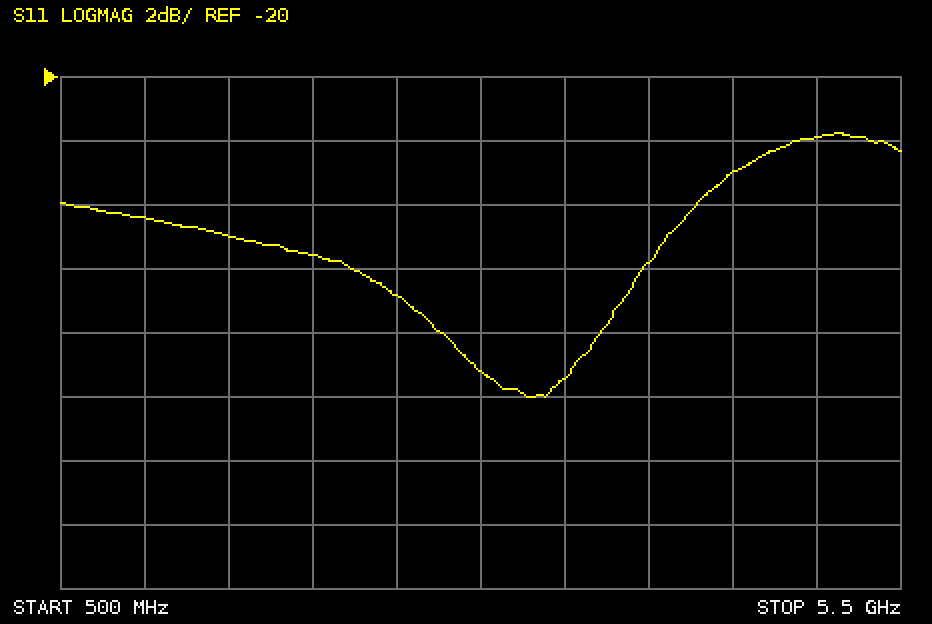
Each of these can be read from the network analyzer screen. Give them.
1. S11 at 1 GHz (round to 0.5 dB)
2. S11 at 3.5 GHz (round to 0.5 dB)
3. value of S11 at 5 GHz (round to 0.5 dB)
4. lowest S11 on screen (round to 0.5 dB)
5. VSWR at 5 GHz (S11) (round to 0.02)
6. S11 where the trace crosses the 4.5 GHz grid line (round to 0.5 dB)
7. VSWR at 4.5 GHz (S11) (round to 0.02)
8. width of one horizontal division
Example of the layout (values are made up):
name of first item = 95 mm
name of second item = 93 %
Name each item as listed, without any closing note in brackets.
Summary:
S11 at 1 GHz = -24.5 dB
S11 at 3.5 GHz = -29.5 dB
value of S11 at 5 GHz = -22.0 dB
lowest S11 on screen = -30.0 dB
VSWR at 5 GHz (S11) = 1.18
S11 where the trace crosses the 4.5 GHz grid line = -23.0 dB
VSWR at 4.5 GHz (S11) = 1.16
width of one horizontal division = 500 MHz
